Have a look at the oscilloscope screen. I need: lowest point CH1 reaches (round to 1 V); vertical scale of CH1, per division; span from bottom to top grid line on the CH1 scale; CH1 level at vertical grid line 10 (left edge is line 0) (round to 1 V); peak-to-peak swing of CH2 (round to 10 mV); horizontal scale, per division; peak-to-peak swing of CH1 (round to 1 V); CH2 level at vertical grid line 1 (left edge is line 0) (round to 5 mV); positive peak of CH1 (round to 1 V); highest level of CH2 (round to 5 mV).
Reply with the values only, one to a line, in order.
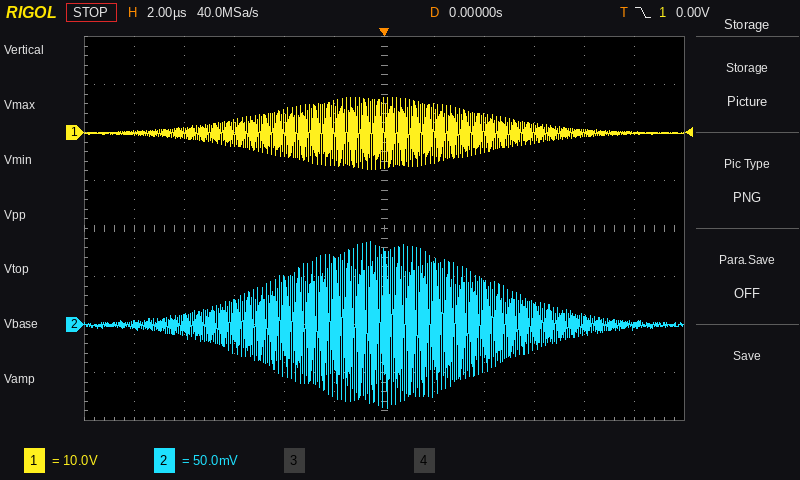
-8 V
10 V
80 V
0 V
170 mV
2 µs
15 V
0 mV
7 V
85 mV
